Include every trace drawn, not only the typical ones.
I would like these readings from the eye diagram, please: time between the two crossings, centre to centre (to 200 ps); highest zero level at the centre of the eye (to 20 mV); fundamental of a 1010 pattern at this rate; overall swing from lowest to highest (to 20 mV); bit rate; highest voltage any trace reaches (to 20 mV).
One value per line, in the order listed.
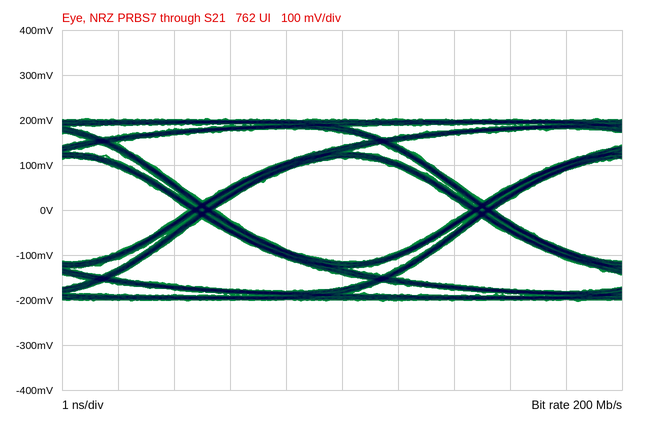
5.0 ns
-120 mV
100 MHz
400 mV
200 Mb/s
200 mV
